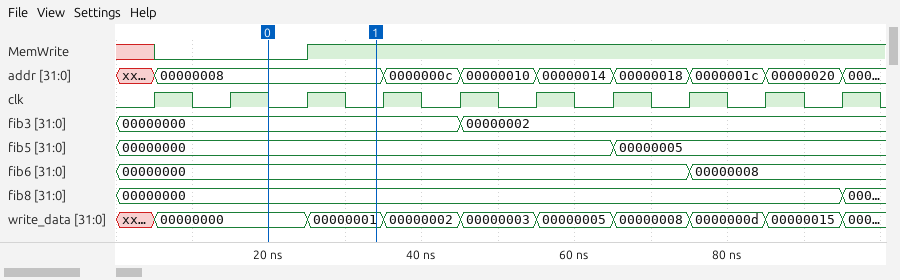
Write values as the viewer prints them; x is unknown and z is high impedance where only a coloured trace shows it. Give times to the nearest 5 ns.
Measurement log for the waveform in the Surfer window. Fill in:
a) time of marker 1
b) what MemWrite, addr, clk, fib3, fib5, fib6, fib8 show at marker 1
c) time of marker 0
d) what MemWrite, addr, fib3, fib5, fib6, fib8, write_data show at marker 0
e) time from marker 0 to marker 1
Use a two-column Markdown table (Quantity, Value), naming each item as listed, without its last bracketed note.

| Quantity | Value |
|---|---|
| time of marker 1 | 35 ns |
| what MemWrite, addr, clk, fib3, fib5, fib6, fib8 show at marker 1 | MemWrite=1, addr=00000008, clk=0, fib3=00000000, fib5=00000000, fib6=00000000, fib8=00000000 |
| time of marker 0 | 20 ns |
| what MemWrite, addr, fib3, fib5, fib6, fib8, write_data show at marker 0 | MemWrite=0, addr=00000008, fib3=00000000, fib5=00000000, fib6=00000000, fib8=00000000, write_data=00000000 |
| time from marker 0 to marker 1 | 15 ns |
